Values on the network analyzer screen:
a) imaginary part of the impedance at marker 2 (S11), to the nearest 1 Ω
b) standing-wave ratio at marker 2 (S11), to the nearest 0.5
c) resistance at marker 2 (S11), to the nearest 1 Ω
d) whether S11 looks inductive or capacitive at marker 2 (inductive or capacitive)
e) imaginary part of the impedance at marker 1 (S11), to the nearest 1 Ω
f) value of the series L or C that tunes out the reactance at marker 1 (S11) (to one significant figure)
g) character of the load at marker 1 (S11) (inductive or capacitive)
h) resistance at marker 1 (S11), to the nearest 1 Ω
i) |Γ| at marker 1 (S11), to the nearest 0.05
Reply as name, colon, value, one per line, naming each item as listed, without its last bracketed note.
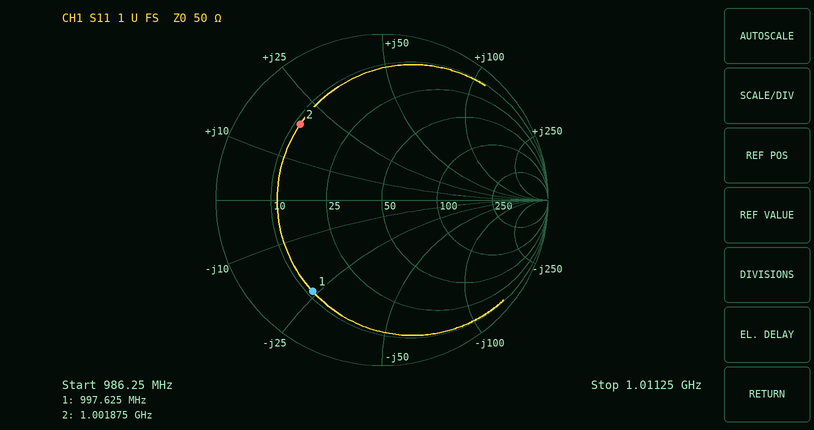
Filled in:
imaginary part of the impedance at marker 2 (S11), to the nearest 1 Ω: +19 Ω
standing-wave ratio at marker 2 (S11), to the nearest 0.5: 5.0
resistance at marker 2 (S11), to the nearest 1 Ω: 11 Ω
whether S11 looks inductive or capacitive at marker 2: inductive
imaginary part of the impedance at marker 1 (S11), to the nearest 1 Ω: -24 Ω
value of the series L or C that tunes out the reactance at marker 1 (S11): 4 nH
character of the load at marker 1 (S11): capacitive
resistance at marker 1 (S11), to the nearest 1 Ω: 11 Ω
|Γ| at marker 1 (S11), to the nearest 0.05: 0.70
